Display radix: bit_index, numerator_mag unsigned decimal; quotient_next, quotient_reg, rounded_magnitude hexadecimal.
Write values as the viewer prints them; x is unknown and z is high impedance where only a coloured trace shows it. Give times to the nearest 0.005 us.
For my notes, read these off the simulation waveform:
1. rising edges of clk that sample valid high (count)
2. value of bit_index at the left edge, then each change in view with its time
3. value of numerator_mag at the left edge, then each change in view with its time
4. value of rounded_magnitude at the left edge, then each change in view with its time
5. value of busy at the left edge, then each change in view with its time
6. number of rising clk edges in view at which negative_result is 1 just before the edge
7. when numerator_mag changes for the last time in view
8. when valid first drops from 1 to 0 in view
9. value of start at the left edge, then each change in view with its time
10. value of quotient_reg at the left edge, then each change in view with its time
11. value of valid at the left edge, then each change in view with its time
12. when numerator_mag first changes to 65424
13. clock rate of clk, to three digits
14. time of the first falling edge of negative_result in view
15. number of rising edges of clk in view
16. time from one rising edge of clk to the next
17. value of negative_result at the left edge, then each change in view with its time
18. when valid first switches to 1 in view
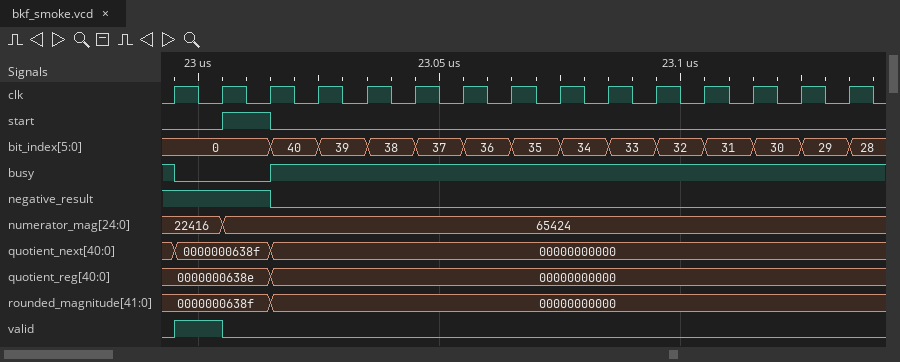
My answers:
1
0, 40 at 23.015 us, 39 at 23.025 us, 38 at 23.035 us, 37 at 23.045 us, 36 at 23.055 us, 35 at 23.065 us, 34 at 23.075 us, 33 at 23.085 us, 32 at 23.095 us, 31 at 23.105 us, 30 at 23.115 us, 29 at 23.125 us, 28 at 23.135 us
22416, 65424 at 23.005 us
0000000638f, 00000000000 at 23.015 us
1, 0 at 22.995 us, 1 at 23.015 us
3
23.005 us
23.005 us
0, 1 at 23.005 us, 0 at 23.015 us
0000000638e, 00000000000 at 23.015 us
0, 1 at 22.995 us, 0 at 23.005 us
23.005 us
100 MHz
23.015 us
15
0.01 us
1, 0 at 23.015 us
22.995 us
